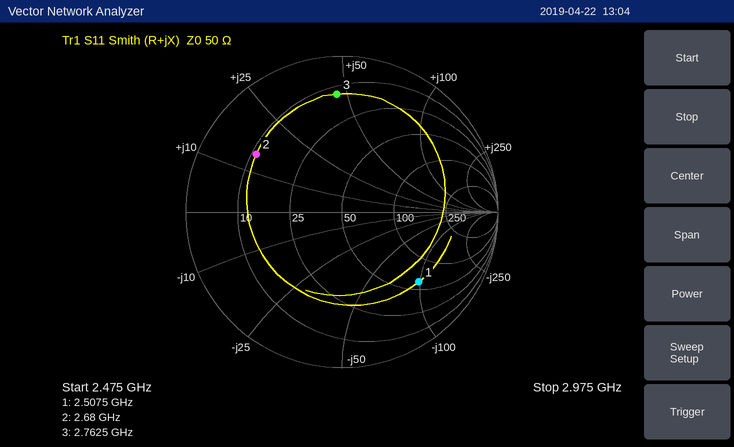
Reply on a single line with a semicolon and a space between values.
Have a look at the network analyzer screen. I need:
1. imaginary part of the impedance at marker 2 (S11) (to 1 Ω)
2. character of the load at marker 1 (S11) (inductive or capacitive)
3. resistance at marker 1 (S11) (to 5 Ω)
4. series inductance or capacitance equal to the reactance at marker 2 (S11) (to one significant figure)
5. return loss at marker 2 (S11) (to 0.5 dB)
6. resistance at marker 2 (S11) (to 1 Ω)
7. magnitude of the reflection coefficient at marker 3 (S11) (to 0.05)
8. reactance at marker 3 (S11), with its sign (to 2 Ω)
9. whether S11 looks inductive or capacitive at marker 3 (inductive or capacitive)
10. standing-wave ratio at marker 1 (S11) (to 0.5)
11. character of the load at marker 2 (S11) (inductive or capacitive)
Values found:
+15 Ω; capacitive; 60 Ω; 900 pH; 3.5 dB; 11 Ω; 0.75; +46 Ω; inductive; 5.0; inductive
